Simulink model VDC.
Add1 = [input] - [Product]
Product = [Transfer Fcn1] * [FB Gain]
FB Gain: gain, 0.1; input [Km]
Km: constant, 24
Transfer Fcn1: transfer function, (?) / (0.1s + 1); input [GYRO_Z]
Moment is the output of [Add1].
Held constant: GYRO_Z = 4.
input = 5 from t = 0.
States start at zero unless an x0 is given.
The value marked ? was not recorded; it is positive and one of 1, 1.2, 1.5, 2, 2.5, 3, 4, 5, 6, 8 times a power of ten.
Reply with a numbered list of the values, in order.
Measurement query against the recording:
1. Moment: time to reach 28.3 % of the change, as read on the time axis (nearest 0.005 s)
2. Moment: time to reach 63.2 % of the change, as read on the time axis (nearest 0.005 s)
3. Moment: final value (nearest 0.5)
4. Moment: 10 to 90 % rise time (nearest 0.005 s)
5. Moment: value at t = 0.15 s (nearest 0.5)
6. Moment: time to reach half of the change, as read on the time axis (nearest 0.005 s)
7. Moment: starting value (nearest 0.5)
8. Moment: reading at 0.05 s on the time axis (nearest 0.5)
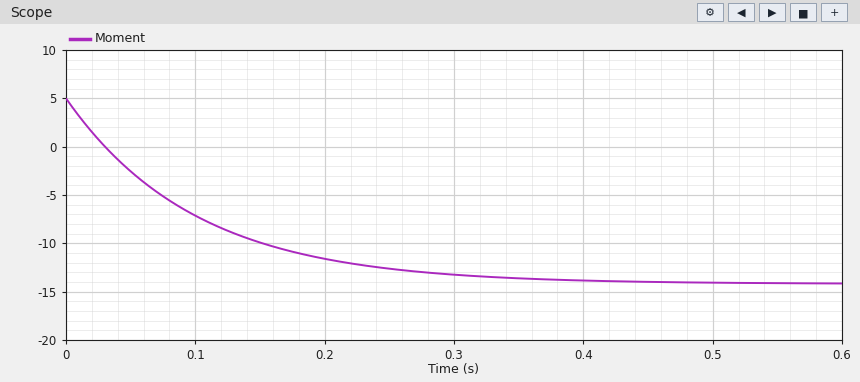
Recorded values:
1. 0.035 s
2. 0.100 s
3. -14.0
4. 0.220 s
5. -10.0
6. 0.070 s
7. 5.0
8. -2.5
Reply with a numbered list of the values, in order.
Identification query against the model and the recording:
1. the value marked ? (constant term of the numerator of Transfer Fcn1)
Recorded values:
1. 2
